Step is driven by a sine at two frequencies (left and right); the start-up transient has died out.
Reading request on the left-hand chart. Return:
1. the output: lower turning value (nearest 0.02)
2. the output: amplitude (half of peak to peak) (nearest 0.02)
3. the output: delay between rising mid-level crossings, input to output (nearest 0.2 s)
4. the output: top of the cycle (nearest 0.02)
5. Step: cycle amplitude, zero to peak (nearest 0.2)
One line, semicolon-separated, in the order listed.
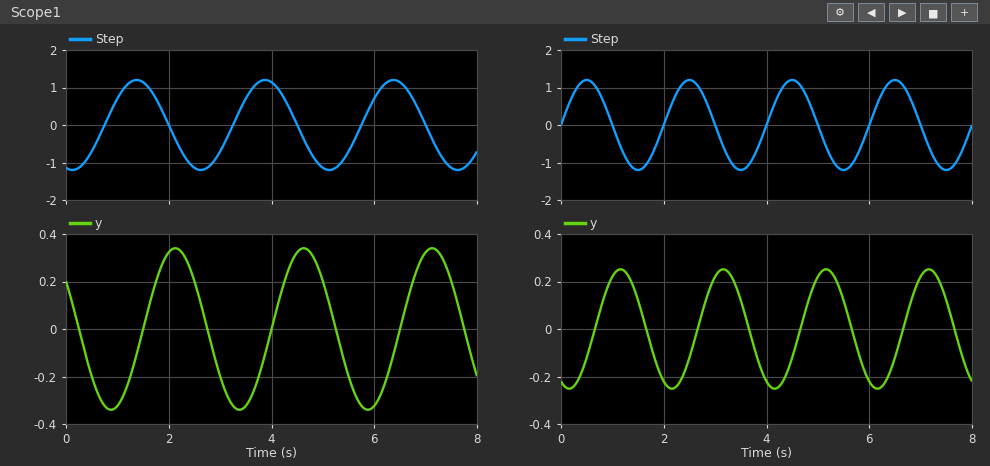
-0.34; 0.34; 0.8 s; 0.34; 1.2
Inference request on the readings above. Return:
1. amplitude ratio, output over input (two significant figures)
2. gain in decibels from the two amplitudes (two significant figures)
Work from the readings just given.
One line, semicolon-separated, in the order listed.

0.28; -11 dB
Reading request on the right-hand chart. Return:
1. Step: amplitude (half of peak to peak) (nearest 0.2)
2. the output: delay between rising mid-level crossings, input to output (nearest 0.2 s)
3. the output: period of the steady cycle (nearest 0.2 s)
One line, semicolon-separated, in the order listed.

1.2; 0.6 s; 2.0 s
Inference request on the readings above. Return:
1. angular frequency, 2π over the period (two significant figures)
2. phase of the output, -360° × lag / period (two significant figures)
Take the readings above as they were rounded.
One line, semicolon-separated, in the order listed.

3.1 rad/s; -110°
